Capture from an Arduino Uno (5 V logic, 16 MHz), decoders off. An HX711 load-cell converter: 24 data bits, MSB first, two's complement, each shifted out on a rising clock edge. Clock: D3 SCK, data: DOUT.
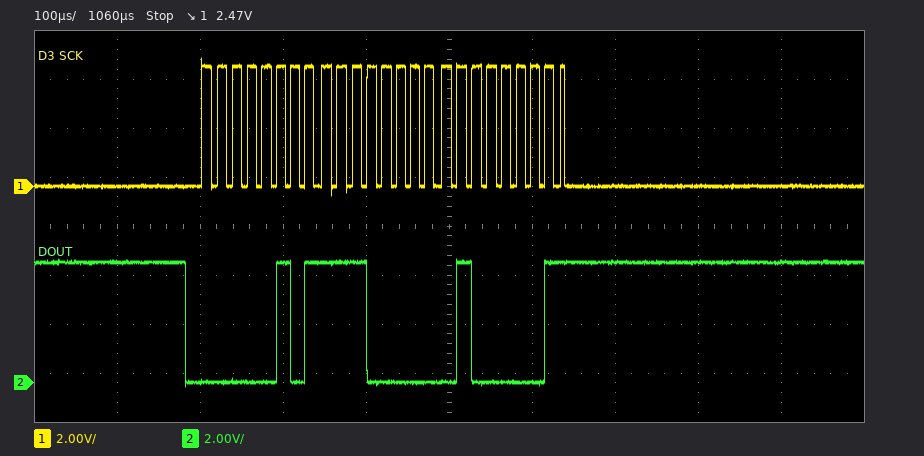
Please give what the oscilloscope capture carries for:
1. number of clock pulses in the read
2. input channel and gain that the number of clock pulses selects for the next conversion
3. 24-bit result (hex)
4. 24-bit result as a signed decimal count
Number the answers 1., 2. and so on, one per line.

1. 25
2. channel A, gain 128
3. 0x05E041
4. 385089
